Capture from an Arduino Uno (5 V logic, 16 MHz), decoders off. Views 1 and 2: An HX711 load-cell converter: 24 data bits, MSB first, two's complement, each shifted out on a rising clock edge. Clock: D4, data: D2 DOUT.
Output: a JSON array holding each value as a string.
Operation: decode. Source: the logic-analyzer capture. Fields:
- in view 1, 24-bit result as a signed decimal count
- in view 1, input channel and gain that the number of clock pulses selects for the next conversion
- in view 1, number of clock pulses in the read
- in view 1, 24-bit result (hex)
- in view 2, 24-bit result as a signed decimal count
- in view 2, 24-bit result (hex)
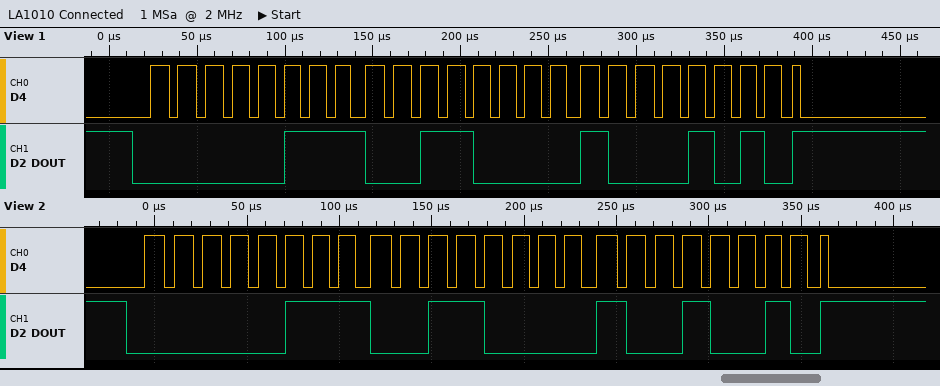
["471178", "channel A, gain 128", "25", "0x07308A", "471186", "0x073092"]
